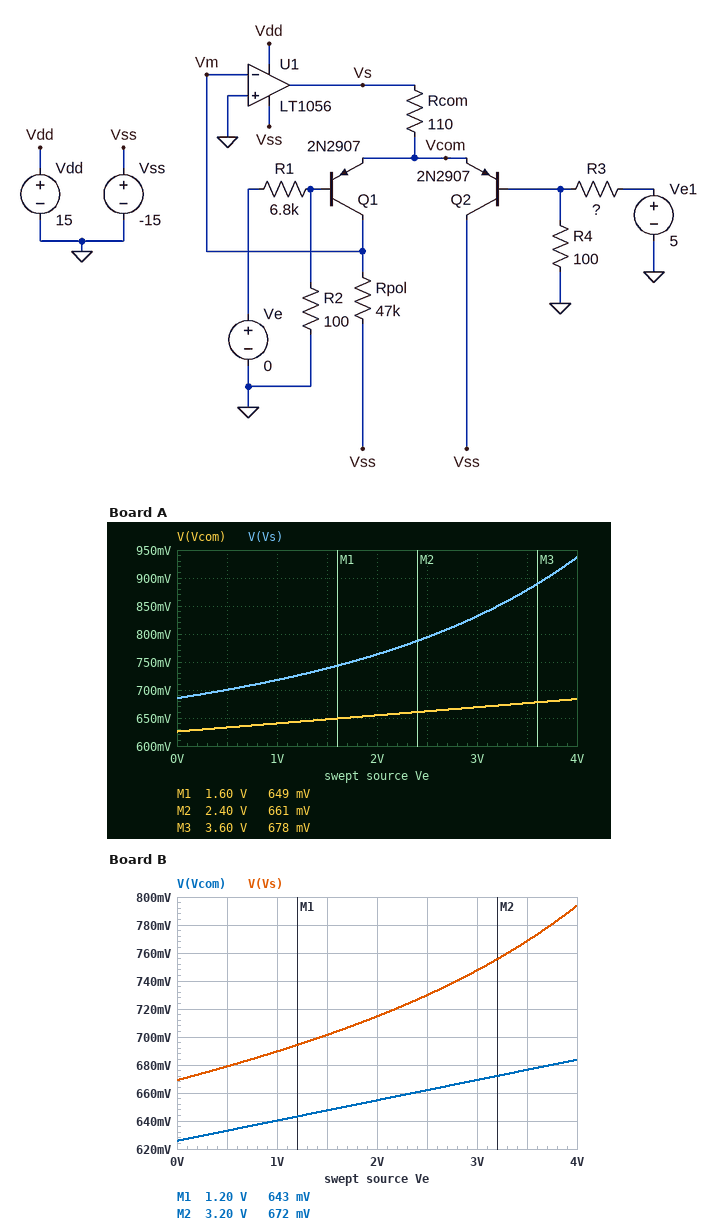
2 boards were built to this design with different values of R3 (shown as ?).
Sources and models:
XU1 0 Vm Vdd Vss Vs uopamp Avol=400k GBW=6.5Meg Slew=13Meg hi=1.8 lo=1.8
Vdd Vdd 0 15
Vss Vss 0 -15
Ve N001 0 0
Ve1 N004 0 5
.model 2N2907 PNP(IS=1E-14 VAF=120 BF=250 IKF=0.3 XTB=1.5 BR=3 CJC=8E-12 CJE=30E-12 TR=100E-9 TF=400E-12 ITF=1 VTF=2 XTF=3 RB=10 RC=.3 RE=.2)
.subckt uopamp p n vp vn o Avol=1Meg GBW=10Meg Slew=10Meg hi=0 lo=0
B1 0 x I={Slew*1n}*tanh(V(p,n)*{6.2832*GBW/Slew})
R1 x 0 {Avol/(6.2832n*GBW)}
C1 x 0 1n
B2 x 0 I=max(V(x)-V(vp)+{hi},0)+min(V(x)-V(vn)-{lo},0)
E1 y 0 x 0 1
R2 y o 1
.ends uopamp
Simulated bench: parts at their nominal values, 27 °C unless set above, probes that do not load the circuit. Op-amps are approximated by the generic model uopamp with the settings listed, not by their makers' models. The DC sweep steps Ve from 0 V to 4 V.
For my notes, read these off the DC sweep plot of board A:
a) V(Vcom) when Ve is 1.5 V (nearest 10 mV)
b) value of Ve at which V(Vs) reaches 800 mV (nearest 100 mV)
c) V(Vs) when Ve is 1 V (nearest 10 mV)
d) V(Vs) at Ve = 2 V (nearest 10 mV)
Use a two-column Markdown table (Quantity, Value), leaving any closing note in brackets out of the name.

| Quantity | Value |
|---|---|
| V(Vcom) when Ve is 1.5 V | 650 mV |
| value of Ve at which V(Vs) reaches 800 mV | 2.6 V |
| V(Vs) when Ve is 1 V | 720 mV |
| V(Vs) at Ve = 2 V | 760 mV |
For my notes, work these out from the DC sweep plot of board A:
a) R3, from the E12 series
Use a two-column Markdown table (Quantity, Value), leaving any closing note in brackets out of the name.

| Quantity | Value |
|---|---|
| R3, from the E12 series | 39 kΩ |
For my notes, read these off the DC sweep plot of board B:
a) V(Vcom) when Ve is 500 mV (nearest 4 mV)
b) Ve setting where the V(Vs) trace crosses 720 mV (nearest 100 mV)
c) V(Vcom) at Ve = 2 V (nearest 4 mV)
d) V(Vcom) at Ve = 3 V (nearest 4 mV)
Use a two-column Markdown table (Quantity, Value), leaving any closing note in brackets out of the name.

| Quantity | Value |
|---|---|
| V(Vcom) when Ve is 500 mV | 632 mV |
| Ve setting where the V(Vs) trace crosses 720 mV | 2.2 V |
| V(Vcom) at Ve = 2 V | 656 mV |
| V(Vcom) at Ve = 3 V | 668 mV |
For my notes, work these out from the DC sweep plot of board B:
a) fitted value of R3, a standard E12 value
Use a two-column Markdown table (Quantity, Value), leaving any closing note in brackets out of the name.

| Quantity | Value |
|---|---|
| fitted value of R3, a standard E12 value | 12 kΩ |
